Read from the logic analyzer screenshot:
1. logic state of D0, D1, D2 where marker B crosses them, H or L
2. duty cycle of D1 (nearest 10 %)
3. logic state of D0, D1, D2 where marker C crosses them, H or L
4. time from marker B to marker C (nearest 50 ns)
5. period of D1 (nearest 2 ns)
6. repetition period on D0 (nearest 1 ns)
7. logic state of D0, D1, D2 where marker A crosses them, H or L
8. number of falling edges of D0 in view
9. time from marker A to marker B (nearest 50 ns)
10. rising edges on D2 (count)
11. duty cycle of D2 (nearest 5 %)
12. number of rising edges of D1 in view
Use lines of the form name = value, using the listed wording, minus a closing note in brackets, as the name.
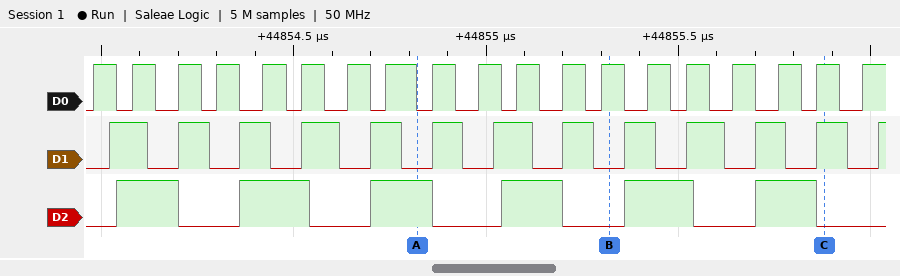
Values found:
logic state of D0, D1, D2 where marker B crosses them, H or L = D0=H, D1=L, D2=L
duty cycle of D1 = 50 %
logic state of D0, D1, D2 where marker C crosses them, H or L = D0=H, D1=H, D2=L
time from marker B to marker C = 550 ns
period of D1 = 166 ns
repetition period on D0 = 111 ns
logic state of D0, D1, D2 where marker A crosses them, H or L = D0=L, D1=L, D2=H
number of falling edges of D0 in view = 18
time from marker A to marker B = 500 ns
rising edges on D2 = 6
duty cycle of D2 = 50 %
number of rising edges of D1 in view = 13
